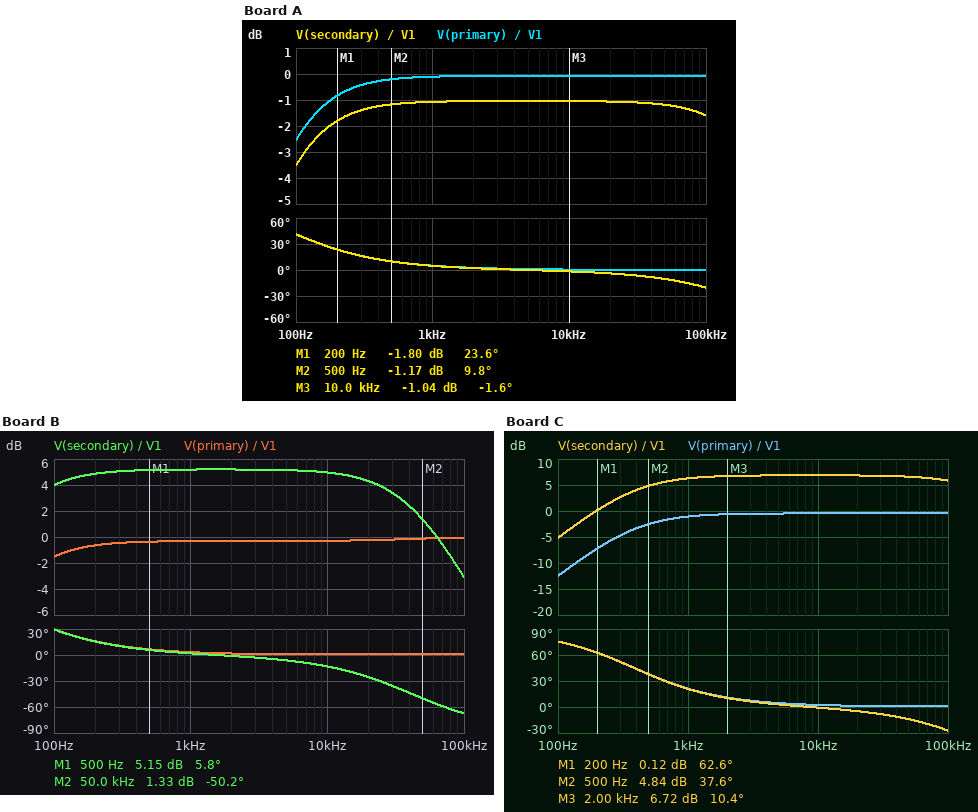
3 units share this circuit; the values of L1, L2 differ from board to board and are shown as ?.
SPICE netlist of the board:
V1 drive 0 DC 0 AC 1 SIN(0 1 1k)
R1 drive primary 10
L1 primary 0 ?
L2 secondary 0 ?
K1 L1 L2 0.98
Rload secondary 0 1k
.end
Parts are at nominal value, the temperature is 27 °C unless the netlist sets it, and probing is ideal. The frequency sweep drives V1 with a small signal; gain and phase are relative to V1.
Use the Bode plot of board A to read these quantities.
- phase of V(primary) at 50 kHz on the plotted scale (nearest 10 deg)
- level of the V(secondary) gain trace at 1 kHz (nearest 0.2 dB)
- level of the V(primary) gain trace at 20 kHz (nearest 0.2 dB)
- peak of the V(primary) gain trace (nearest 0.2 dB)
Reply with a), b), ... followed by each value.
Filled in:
a) 0 deg
b) -1.0 dB
c) 0 dB
d) 0 dB
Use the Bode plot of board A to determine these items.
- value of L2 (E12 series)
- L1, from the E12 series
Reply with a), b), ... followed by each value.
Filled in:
a) 15 mH
b) 18 mH
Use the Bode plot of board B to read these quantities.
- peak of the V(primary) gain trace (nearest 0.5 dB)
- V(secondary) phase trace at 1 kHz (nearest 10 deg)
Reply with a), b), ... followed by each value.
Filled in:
a) 0 dB
b) 0 deg
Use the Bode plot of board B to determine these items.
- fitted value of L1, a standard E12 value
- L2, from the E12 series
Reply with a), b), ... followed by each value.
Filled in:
a) 27 mH
b) 100 mH
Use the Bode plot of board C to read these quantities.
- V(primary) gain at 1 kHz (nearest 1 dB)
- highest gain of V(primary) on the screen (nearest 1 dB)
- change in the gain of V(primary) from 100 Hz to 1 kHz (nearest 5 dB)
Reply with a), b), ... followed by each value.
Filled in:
a) -1 dB
b) 0 dB
c) 10 dB
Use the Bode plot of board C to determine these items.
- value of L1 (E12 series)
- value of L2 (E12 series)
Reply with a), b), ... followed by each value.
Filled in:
a) 3.9 mH
b) 22 mH
